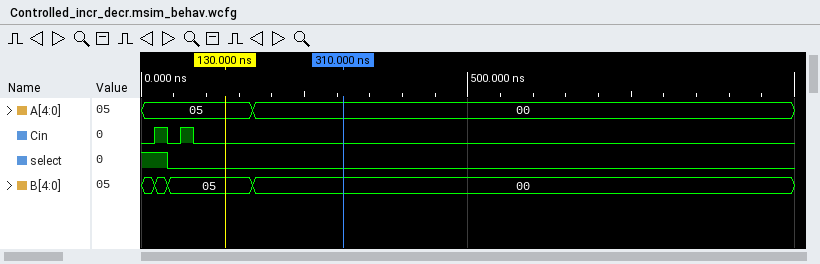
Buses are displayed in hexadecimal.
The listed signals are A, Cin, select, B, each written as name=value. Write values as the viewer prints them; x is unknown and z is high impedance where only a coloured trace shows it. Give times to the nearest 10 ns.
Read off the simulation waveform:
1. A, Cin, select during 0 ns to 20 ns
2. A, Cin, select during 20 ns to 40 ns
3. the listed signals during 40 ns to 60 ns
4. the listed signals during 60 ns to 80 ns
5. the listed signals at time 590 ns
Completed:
A=05, Cin=0, select=1
A=05, Cin=1, select=1
A=05, Cin=0, select=0, B=05
A=05, Cin=1, select=0, B=05
A=00, Cin=0, select=0, B=00
